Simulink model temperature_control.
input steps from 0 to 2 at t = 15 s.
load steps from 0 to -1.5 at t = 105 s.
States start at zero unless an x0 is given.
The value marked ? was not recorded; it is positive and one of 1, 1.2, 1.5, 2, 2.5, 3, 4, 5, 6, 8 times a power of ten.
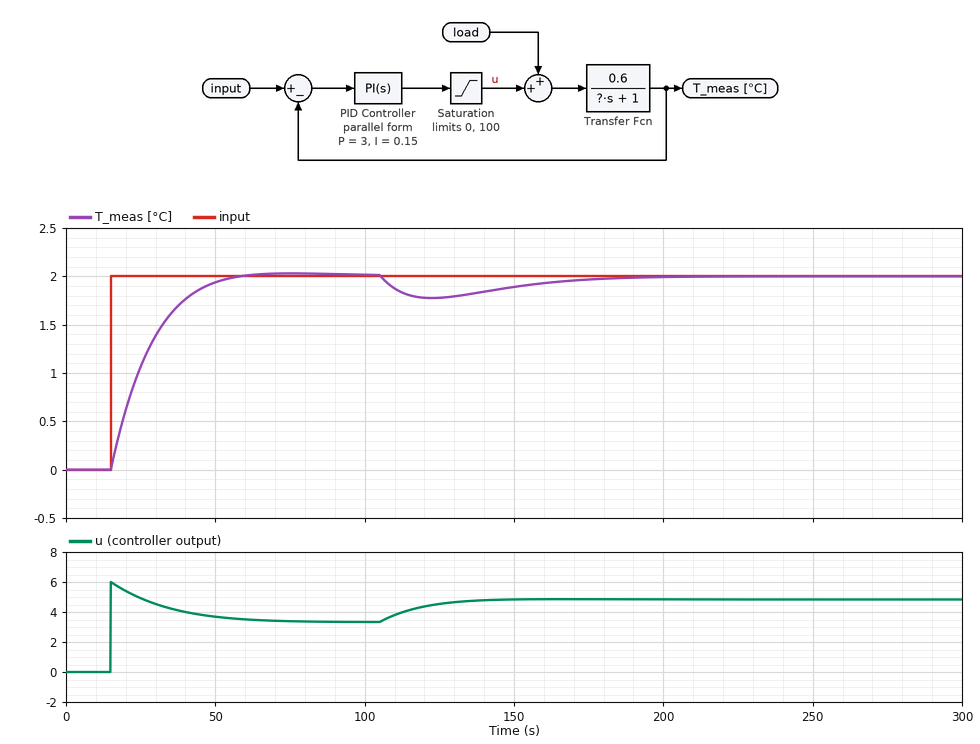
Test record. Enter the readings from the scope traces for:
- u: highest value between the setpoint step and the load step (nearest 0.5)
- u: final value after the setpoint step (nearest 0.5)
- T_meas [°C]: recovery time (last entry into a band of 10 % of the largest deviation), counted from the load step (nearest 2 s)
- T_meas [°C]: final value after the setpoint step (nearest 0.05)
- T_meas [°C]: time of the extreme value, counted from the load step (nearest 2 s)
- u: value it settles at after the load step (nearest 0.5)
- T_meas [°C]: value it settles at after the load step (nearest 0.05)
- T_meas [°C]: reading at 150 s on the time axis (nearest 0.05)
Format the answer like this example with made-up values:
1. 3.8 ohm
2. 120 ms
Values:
1. 6.0
2. 3.5
3. 76 s
4. 2.00
5. 18 s
6. 5.0
7. 2.00
8. 1.90
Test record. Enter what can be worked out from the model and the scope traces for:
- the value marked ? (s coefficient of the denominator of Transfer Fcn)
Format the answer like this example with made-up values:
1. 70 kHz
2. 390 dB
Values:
1. 25
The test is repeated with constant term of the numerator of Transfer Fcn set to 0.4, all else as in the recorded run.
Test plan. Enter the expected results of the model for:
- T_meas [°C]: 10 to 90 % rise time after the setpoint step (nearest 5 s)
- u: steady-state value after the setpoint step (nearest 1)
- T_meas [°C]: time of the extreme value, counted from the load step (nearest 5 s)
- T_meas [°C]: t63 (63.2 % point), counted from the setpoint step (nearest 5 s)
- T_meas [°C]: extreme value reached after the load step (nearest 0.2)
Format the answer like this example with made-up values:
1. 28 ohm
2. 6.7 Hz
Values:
1. 35 s
2. 5
3. 20 s
4. 20 s
5. 1.8
